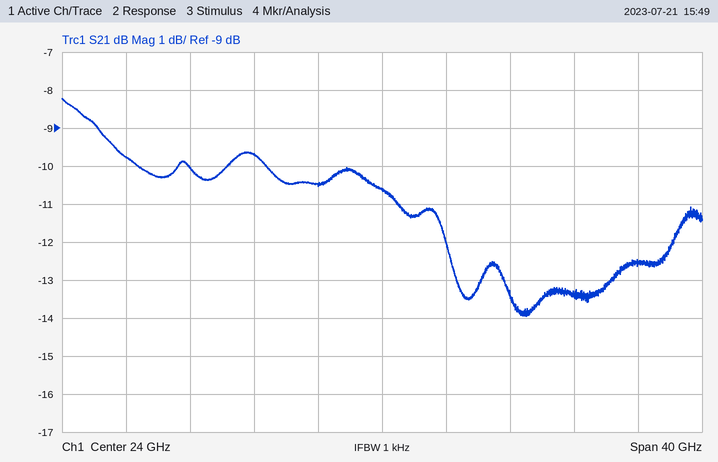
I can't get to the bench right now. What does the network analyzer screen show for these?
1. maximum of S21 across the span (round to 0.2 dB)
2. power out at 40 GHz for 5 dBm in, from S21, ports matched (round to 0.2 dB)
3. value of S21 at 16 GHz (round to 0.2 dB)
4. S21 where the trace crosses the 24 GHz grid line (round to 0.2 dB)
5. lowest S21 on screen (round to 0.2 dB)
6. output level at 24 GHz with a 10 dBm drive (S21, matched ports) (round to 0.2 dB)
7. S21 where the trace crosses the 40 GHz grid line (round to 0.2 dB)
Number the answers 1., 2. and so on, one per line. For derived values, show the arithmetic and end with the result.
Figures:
1. -8.2 dB
2. 5 dBm + (-12.6 dB) = -7.6 dBm
3. -9.6 dB
4. -10.6 dB
5. -14.0 dB
6. 10 dBm + (-10.6 dB) = -0.6 dBm
7. -12.6 dB
